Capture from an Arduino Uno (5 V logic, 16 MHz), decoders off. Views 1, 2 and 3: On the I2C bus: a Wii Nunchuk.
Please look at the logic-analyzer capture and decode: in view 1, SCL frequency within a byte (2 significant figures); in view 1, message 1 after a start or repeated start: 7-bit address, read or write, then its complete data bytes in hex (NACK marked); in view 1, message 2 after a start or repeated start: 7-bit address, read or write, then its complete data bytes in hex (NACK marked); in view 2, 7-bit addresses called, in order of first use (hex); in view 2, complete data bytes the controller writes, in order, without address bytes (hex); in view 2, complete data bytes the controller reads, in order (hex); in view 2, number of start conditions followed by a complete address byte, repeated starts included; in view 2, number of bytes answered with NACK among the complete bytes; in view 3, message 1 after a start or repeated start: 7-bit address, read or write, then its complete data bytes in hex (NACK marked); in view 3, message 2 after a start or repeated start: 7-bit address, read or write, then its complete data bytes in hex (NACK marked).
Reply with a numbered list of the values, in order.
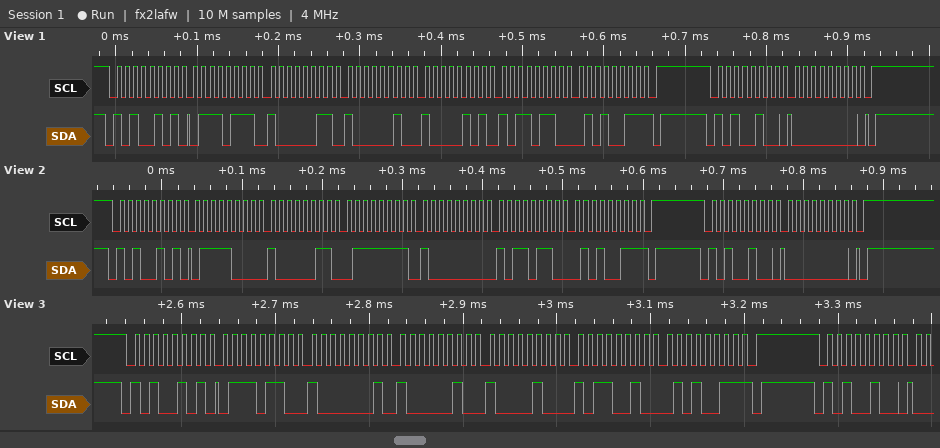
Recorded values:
1. 100 kHz
2. 0x52 read: 77 83 82 85 B6 53 NACK
3. 0x52 write: 00
4. 0x52
5. 00
6. 78 83 7F 80 B6 53
7. 2
8. 1
9. 0x52 read: 76 81 82 84 B2 53 NACK
10. 0x52 write
